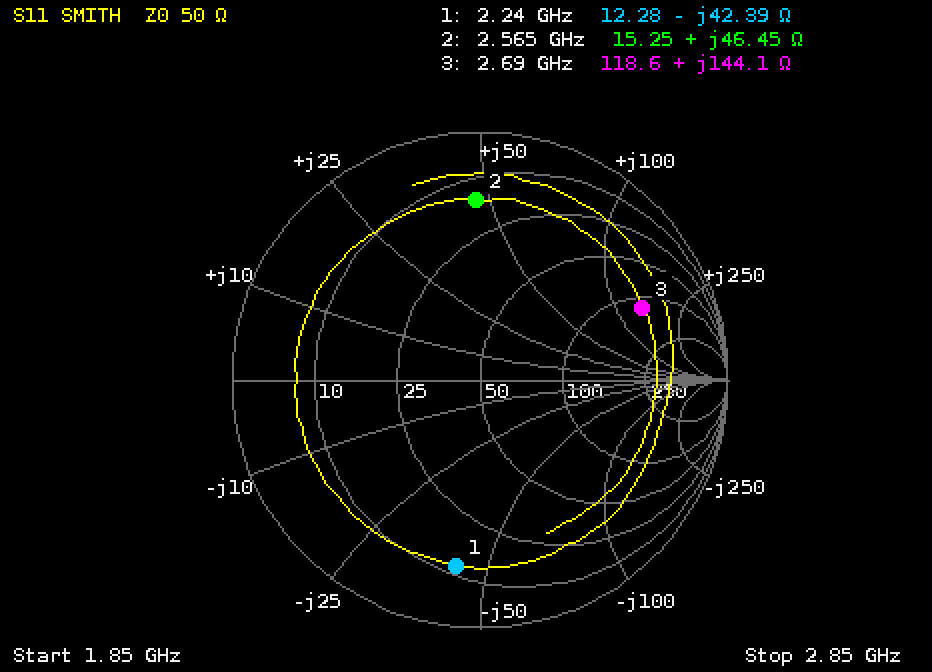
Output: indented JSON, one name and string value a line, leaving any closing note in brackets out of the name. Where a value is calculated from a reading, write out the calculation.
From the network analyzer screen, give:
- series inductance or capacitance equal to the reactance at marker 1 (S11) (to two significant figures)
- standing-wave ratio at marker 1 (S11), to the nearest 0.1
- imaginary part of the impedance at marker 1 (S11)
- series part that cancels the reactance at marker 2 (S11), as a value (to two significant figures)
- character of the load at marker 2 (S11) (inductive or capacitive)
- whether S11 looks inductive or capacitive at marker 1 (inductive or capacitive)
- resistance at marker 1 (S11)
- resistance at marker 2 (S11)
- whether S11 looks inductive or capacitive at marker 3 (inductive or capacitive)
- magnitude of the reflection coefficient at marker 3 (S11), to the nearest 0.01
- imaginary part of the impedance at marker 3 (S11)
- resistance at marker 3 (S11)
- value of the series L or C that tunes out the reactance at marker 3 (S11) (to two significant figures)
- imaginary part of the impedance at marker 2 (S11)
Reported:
{
  "series inductance or capacitance equal to the reactance at marker 1 (S11)": "C = 1/(2π × 2.24 GHz × 42.39 Ω) ≈ 1.7 pF",
  "standing-wave ratio at marker 1 (S11), to the nearest 0.1": "7.1",
  "imaginary part of the impedance at marker 1": "-42.39 Ω",
  "series part that cancels the reactance at marker 2 (S11), as a value": "C = 1/(2π × 2.565 GHz × 46.45 Ω) ≈ 1.3 pF",
  "character of the load at marker 2 (S11)": "inductive",
  "whether S11 looks inductive or capacitive at marker 1": "capacitive",
  "resistance at marker 1": "12.28 Ω",
  "resistance at marker 2": "15.25 Ω",
  "whether S11 looks inductive or capacitive at marker 3": "inductive",
  "magnitude of the reflection coefficient at marker 3 (S11), to the nearest 0.01": "0.72",
  "imaginary part of the impedance at marker 3": "+144.1 Ω",
  "resistance at marker 3": "118.6 Ω",
  "value of the series L or C that tunes out the reactance at marker 3 (S11)": "C = 1/(2π × 2.69 GHz × 144.1 Ω) ≈ 411 fF, so 410 fF to two significant figures",
  "imaginary part of the impedance at marker 2": "+46.45 Ω"
}
